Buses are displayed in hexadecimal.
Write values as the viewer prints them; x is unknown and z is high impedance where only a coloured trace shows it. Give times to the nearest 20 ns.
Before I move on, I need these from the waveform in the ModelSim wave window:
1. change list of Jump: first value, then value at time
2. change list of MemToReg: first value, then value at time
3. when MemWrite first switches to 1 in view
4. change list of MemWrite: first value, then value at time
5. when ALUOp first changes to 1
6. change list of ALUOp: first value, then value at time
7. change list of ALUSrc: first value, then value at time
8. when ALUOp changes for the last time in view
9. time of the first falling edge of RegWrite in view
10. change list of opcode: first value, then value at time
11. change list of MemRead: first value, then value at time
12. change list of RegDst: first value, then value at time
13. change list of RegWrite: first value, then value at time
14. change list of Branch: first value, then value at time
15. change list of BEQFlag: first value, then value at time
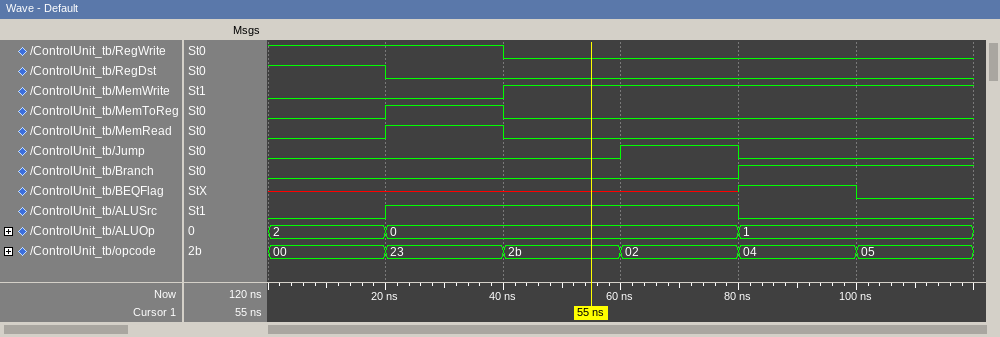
0, 1 at 60 ns, 0 at 80 ns
0, 1 at 20 ns, 0 at 40 ns
40 ns
0, 1 at 40 ns
80 ns
2, 0 at 20 ns, 1 at 80 ns
0, 1 at 20 ns, 0 at 80 ns
80 ns
40 ns
00, 23 at 20 ns, 2b at 40 ns, 02 at 60 ns, 04 at 80 ns, 05 at 100 ns
0, 1 at 20 ns, 0 at 40 ns
1, 0 at 20 ns
1, 0 at 40 ns
0, 1 at 80 ns
x, 1 at 80 ns, 0 at 100 ns
